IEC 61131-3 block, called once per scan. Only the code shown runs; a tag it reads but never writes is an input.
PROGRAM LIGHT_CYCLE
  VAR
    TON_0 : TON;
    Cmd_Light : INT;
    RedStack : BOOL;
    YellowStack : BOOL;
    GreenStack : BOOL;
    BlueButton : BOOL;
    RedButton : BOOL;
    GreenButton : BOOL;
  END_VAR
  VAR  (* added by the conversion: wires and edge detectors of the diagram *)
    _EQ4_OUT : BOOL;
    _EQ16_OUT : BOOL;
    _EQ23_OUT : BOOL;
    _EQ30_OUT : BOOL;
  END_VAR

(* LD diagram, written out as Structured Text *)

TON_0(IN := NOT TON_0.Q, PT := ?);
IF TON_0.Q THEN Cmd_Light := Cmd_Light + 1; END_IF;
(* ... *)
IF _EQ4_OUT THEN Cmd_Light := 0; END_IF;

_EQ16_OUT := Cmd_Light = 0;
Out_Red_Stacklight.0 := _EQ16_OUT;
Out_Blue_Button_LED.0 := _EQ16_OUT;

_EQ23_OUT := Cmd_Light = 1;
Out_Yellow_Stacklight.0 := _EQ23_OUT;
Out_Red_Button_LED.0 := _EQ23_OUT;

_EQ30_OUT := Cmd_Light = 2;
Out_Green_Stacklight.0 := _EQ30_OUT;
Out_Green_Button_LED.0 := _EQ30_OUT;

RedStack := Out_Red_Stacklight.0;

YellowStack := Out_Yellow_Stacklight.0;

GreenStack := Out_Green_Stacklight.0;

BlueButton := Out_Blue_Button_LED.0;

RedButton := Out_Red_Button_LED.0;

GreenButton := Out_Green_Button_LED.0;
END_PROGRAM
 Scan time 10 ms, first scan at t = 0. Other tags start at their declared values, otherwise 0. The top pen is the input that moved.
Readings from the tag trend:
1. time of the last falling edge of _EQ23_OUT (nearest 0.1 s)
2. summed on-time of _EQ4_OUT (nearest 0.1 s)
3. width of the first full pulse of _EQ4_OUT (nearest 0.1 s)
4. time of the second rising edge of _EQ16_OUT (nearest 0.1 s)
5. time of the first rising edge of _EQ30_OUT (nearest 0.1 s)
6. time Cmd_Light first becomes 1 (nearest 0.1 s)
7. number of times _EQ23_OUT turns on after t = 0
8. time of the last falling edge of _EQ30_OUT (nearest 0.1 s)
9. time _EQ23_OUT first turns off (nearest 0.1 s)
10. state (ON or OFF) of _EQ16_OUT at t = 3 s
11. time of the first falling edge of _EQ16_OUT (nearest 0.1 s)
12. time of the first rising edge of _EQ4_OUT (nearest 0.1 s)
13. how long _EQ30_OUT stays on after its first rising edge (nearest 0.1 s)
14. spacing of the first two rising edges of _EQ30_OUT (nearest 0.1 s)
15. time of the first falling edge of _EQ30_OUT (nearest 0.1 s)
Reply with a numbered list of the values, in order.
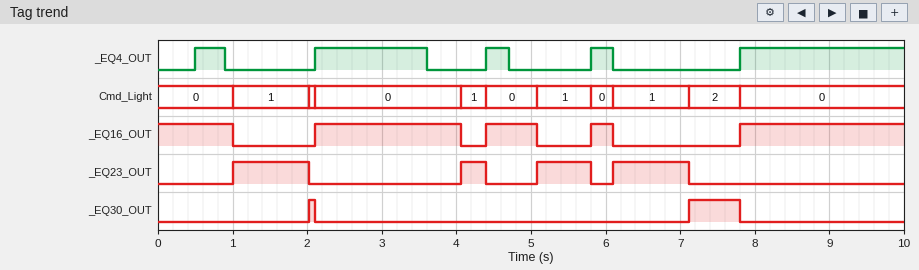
1. 7.1 s
2. 4.7 s
3. 0.4 s
4. 4.4 s
5. 2.0 s
6. 1.0 s
7. 4
8. 7.8 s
9. 2.0 s
10. ON
11. 1.0 s
12. 0.5 s
13. 0.1 s
14. 5.1 s
15. 2.1 s
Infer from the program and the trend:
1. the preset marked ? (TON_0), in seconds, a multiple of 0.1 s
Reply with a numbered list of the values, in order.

1. 1.0 s
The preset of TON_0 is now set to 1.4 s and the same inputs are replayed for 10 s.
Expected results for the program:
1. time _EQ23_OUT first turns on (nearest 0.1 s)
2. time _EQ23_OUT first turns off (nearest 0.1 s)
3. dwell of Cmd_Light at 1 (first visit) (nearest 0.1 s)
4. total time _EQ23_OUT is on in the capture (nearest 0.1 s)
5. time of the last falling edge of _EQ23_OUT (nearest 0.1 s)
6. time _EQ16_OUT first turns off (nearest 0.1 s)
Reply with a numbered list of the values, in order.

1. 1.4 s
2. 2.1 s
3. 0.7 s
4. 1.7 s
5. 7.8 s
6. 1.4 s
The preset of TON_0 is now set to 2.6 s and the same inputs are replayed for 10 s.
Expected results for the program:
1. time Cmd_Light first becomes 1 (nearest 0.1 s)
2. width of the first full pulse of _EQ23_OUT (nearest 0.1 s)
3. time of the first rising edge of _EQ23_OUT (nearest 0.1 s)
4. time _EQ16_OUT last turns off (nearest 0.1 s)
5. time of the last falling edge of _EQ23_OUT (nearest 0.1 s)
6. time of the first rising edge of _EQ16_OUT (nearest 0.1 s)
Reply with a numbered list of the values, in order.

1. 5.2 s
2. 0.6 s
3. 5.2 s
4. 5.2 s
5. 5.8 s
6. 5.8 s
